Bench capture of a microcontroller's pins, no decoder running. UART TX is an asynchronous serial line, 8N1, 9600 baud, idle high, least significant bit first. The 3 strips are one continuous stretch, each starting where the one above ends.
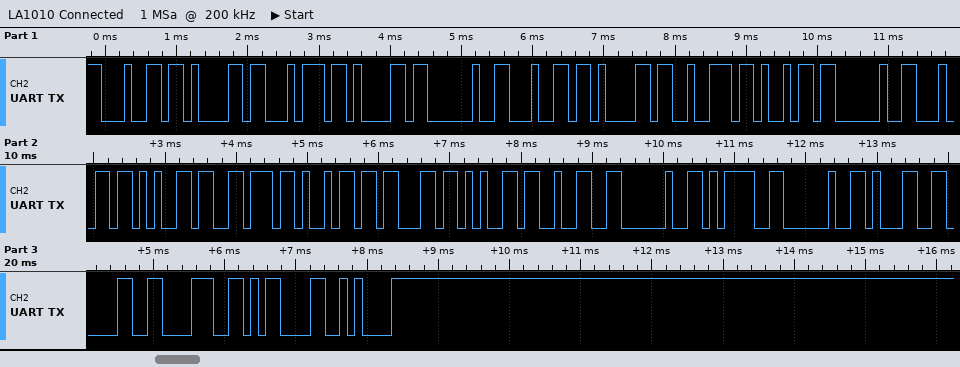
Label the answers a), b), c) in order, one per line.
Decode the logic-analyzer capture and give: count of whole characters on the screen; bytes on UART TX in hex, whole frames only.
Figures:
a) 25
b) 64 61 74 61 20 64 61 72 69 20 64 65 76 69 63 65 32 20 3D 20 31 30 38 0D 0A
